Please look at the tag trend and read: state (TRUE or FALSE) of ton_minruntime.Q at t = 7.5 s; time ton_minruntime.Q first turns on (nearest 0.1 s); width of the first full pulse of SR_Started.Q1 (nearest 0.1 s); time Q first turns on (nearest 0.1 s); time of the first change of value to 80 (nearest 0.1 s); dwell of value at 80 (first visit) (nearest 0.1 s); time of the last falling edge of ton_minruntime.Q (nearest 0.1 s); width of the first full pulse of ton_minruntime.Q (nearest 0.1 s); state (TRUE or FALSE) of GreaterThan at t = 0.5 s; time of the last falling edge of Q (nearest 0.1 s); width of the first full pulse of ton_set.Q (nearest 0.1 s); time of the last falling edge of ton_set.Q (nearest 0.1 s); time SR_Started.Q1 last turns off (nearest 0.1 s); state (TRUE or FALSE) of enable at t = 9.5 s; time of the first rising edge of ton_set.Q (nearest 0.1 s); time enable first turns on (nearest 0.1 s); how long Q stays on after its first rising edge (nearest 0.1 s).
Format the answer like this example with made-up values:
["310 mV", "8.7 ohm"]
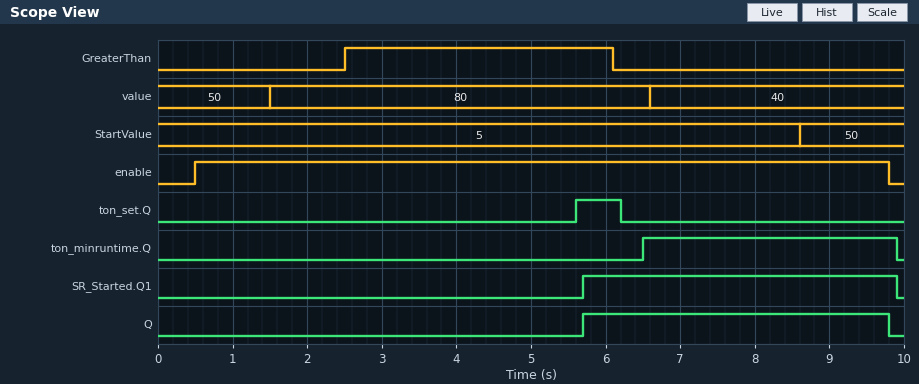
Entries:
["TRUE", "6.5 s", "4.2 s", "5.7 s", "1.5 s", "5.1 s", "9.9 s", "3.4 s", "FALSE", "9.8 s", "0.6 s", "6.2 s", "9.9 s", "TRUE", "5.6 s", "0.5 s", "4.1 s"]
